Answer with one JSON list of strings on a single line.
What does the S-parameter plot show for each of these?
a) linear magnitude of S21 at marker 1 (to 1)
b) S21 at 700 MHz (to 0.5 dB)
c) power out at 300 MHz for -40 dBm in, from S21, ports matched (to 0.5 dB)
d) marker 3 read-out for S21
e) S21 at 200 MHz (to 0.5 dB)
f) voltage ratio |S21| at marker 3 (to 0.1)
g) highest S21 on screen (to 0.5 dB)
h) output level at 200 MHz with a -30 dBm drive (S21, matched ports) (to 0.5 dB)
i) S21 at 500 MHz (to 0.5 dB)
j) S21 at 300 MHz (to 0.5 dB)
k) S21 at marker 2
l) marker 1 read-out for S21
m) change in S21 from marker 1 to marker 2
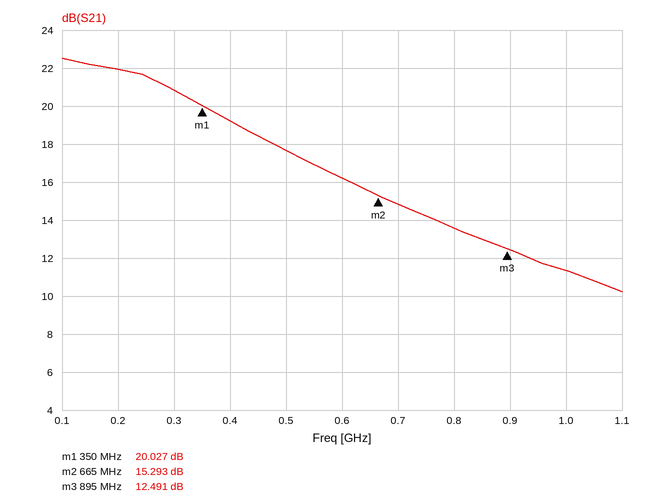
["10", "15.0 dB", "-19.0 dBm", "12.491 dB", "22.0 dB", "4.2", "22.5 dB", "-8.0 dBm", "17.5 dB", "21.0 dB", "15.293 dB", "20.027 dB", "-4.734 dB"]
